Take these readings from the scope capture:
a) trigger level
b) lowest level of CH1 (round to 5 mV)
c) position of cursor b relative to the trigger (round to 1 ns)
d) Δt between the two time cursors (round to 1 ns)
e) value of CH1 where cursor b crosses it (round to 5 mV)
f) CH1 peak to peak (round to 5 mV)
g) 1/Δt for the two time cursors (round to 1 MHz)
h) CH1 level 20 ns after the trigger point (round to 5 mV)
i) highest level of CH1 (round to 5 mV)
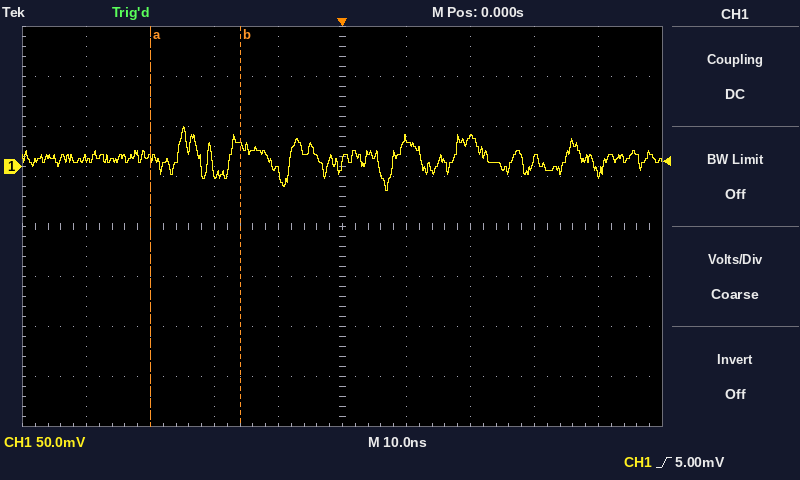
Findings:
5.00 mV
-25 mV
-16 ns
14 ns
20 mV
65 mV
71 MHz
30 mV
40 mV
